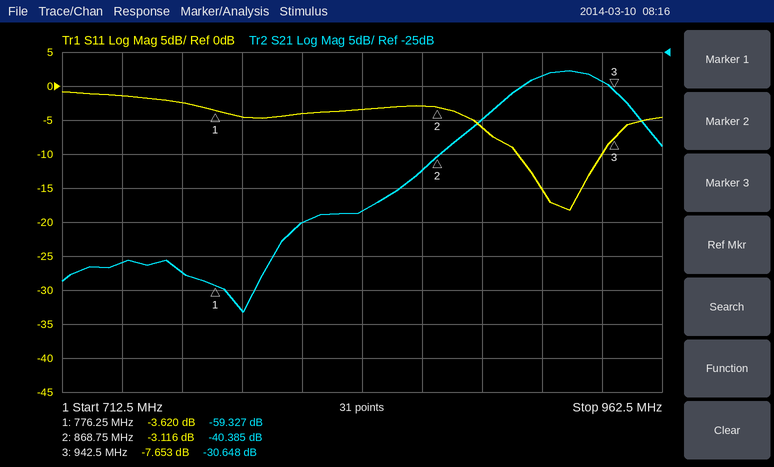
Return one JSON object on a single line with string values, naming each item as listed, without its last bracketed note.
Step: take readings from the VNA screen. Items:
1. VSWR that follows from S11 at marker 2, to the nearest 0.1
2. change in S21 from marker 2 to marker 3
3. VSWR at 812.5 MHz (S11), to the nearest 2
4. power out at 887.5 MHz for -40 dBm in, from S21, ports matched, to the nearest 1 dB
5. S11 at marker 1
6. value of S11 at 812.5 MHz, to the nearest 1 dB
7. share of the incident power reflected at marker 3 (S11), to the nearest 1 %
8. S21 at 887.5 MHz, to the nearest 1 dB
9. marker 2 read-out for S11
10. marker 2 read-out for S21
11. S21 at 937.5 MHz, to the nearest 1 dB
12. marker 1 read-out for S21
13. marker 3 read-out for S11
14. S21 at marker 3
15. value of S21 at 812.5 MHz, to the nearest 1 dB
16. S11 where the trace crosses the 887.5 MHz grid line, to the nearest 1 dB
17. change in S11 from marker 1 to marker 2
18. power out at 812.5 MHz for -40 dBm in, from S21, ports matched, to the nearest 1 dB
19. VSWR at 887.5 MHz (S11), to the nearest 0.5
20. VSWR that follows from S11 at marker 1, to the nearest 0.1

{"VSWR that follows from S11 at marker 2, to the nearest 0.1": "5.6", "change in S21 from marker 2 to marker 3": "9.737 dB", "VSWR at 812.5 MHz (S11), to the nearest 2": "4", "power out at 887.5 MHz for -40 dBm in, from S21, ports matched, to the nearest 1 dB": "-75 dBm", "S11 at marker 1": "-3.620 dB", "value of S11 at 812.5 MHz, to the nearest 1 dB": "-4 dB", "share of the incident power reflected at marker 3 (S11), to the nearest 1 %": "17 %", "S21 at 887.5 MHz, to the nearest 1 dB": "-35 dB", "marker 2 read-out for S11": "-3.116 dB", "marker 2 read-out for S21": "-40.385 dB", "S21 at 937.5 MHz, to the nearest 1 dB": "-29 dB", "marker 1 read-out for S21": "-59.327 dB", "marker 3 read-out for S11": "-7.653 dB", "S21 at marker 3": "-30.648 dB", "value of S21 at 812.5 MHz, to the nearest 1 dB": "-50 dB", "S11 where the trace crosses the 887.5 MHz grid line, to the nearest 1 dB": "-6 dB", "change in S11 from marker 1 to marker 2": "0.504 dB", "power out at 812.5 MHz for -40 dBm in, from S21, ports matched, to the nearest 1 dB": "-90 dBm", "VSWR at 887.5 MHz (S11), to the nearest 0.5": "3.0", "VSWR that follows from S11 at marker 1, to the nearest 0.1": "4.9"}
